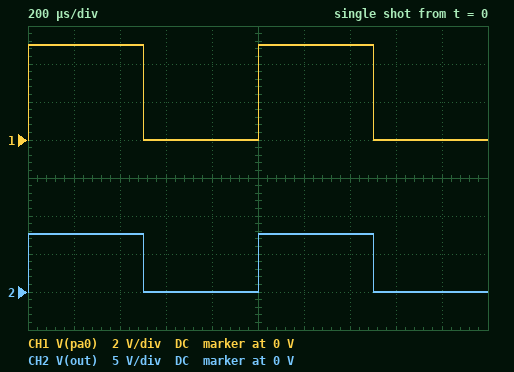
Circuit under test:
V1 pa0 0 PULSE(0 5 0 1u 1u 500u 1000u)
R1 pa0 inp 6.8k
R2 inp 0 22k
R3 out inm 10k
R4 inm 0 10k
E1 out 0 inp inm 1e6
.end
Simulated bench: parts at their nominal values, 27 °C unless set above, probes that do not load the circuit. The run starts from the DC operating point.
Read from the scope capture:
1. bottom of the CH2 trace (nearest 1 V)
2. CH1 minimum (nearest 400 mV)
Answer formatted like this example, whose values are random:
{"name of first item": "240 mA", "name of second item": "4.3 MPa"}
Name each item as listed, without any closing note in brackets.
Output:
{"bottom of the CH2 trace": "0 V", "CH1 minimum": "0 V"}
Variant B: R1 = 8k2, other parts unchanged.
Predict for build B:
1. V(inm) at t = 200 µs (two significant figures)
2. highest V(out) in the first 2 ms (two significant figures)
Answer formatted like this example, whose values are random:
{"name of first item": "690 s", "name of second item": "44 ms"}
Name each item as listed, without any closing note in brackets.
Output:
{"V(inm) at t = 200 µs": "3.6 V", "highest V(out) in the first 2 ms": "7.3 V"}
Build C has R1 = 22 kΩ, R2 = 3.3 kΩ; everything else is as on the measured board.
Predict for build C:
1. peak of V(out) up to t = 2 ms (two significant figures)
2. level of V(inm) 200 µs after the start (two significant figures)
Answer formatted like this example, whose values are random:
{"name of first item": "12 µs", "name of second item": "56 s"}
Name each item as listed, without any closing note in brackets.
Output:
{"peak of V(out) up to t = 2 ms": "1.3 V", "level of V(inm) 200 µs after the start": "650 mV"}
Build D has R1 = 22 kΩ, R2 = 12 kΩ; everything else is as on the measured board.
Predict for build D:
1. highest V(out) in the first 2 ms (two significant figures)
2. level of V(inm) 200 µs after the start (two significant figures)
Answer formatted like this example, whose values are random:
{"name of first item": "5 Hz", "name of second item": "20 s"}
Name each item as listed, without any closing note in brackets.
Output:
{"highest V(out) in the first 2 ms": "3.5 V", "level of V(inm) 200 µs after the start": "1.8 V"}
